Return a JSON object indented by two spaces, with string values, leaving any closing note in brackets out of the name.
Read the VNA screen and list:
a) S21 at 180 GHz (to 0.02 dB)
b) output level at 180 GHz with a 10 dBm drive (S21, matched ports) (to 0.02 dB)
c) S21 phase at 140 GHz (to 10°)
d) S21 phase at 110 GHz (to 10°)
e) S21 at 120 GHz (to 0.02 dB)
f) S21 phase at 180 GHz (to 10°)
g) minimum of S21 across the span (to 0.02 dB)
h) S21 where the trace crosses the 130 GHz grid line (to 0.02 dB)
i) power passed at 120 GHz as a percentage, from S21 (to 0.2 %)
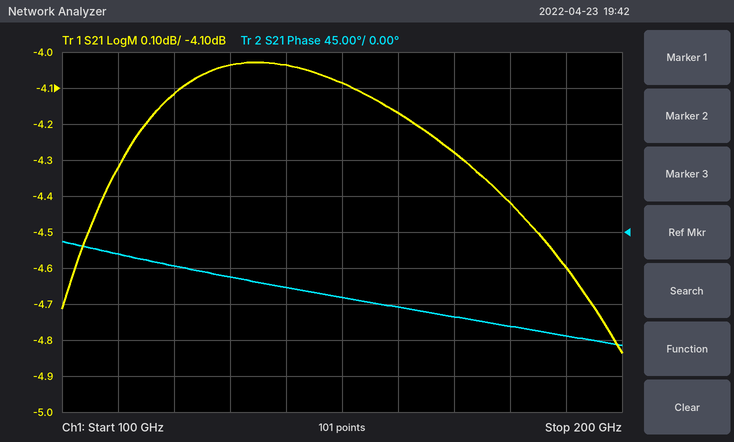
{
  "S21 at 180 GHz": "-4.42 dB",
  "output level at 180 GHz with a 10 dBm drive (S21, matched ports)": "5.58 dBm",
  "S21 phase at 140 GHz": "-70°",
  "S21 phase at 110 GHz": "-30°",
  "S21 at 120 GHz": "-4.12 dB",
  "S21 phase at 180 GHz": "-120°",
  "minimum of S21 across the span": "-4.84 dB",
  "S21 where the trace crosses the 130 GHz grid line": "-4.04 dB",
  "power passed at 120 GHz as a percentage, from S21": "38.8 %"
}
